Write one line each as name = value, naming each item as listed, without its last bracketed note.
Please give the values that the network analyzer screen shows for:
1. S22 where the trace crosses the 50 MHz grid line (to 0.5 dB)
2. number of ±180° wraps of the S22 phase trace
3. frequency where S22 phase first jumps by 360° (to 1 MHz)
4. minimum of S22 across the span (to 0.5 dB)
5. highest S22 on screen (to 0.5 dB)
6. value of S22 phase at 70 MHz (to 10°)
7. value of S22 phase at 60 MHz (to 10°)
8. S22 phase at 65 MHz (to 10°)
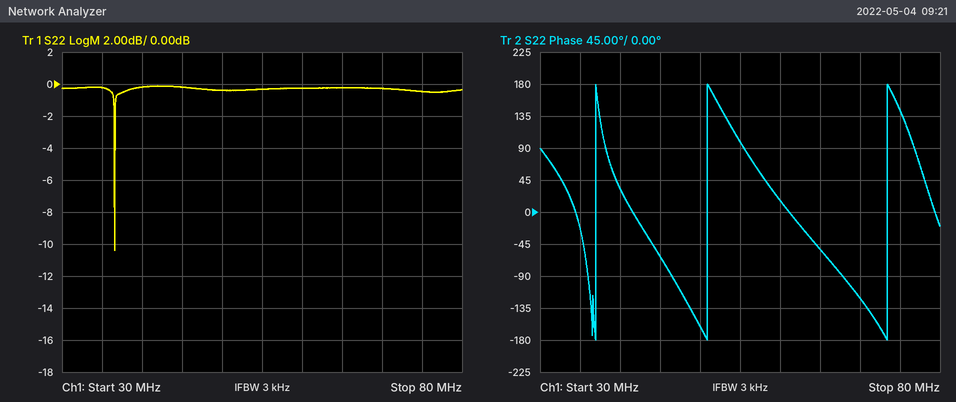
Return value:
S22 where the trace crosses the 50 MHz grid line = -0.5 dB
number of ±180° wraps of the S22 phase trace = 3
frequency where S22 phase first jumps by 360° = 37 MHz
minimum of S22 across the span = -10.5 dB
highest S22 on screen = 0.0 dB
value of S22 phase at 70 MHz = -120°
value of S22 phase at 60 MHz = 20°
S22 phase at 65 MHz = -50°
